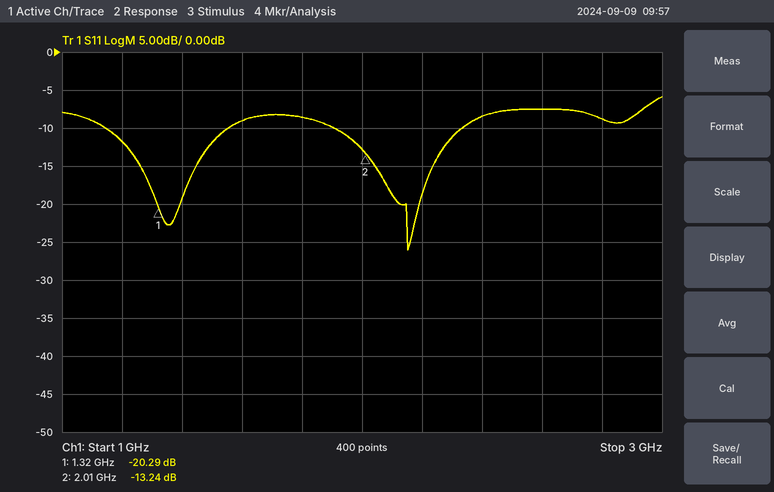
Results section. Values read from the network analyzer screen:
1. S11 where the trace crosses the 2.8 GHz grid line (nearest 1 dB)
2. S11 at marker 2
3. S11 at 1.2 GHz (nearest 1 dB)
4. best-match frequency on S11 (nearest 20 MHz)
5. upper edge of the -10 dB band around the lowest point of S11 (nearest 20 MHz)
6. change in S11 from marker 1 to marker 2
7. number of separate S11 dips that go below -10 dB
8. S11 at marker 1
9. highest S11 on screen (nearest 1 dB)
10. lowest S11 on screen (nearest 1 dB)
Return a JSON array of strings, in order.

["-9 dB", "-13.24 dB", "-12 dB", "2.16 GHz", "2.34 GHz", "7.05 dB", "2", "-20.29 dB", "-6 dB", "-26 dB"]
